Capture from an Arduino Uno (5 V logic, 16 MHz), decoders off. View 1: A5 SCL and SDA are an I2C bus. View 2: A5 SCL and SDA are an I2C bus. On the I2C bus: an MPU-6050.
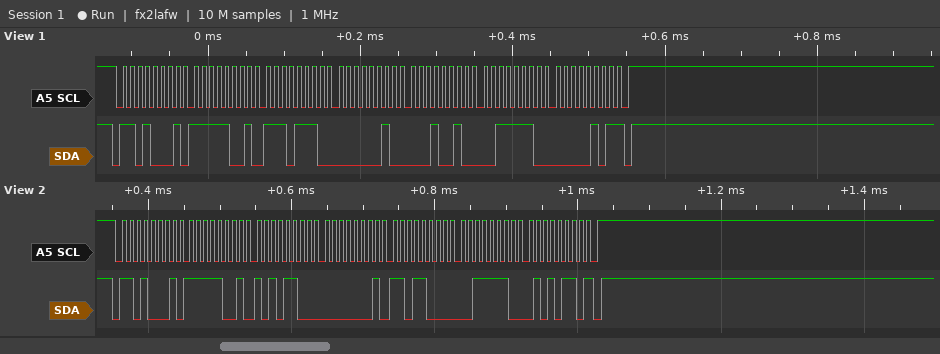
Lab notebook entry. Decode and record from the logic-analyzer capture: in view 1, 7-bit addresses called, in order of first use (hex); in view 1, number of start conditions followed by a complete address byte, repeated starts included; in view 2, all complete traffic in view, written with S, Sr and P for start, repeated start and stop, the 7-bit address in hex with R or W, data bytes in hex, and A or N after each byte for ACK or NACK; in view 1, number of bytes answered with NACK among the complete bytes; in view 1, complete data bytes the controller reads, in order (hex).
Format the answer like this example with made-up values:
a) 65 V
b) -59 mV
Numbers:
a) 0x68
b) 1
c) S 68R A F9 A AC A 01 A D8 A 3E A 56 N P
d) 1
e) F9 EE 02 12 3E 05
